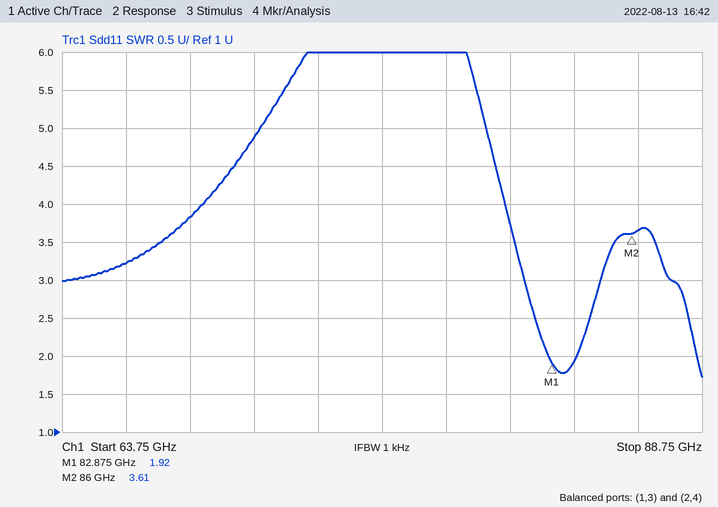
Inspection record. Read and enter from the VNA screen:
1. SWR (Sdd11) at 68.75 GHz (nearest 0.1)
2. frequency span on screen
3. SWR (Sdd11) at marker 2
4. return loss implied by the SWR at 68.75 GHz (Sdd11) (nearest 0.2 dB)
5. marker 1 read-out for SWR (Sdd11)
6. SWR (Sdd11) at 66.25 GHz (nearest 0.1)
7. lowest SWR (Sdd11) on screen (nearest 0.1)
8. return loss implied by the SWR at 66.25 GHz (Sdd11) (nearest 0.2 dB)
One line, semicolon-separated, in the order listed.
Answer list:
3.8; 25 GHz; 3.61; 4.6 dB; 1.92; 3.2; 1.7; 5.6 dB
